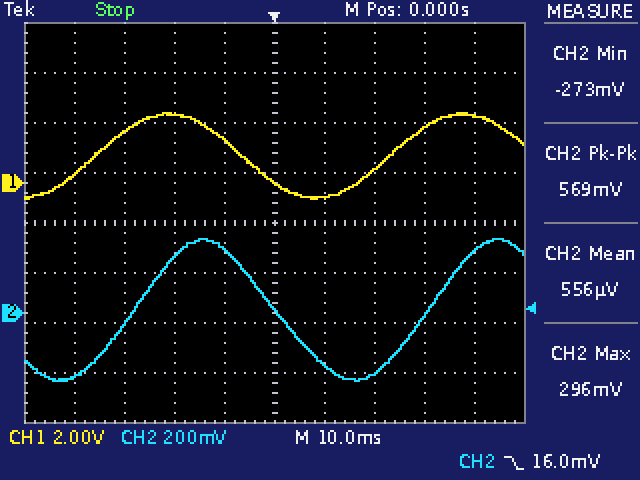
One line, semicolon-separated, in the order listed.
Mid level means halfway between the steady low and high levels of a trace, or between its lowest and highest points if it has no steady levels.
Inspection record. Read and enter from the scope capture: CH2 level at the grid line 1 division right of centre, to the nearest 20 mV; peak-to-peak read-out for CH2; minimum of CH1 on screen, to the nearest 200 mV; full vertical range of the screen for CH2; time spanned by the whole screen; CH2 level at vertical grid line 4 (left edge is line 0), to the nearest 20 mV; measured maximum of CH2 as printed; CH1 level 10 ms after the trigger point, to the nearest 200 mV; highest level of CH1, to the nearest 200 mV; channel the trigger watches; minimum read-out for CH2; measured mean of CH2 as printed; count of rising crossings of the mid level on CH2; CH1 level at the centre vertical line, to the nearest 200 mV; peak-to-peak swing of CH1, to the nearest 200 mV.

-200 mV; 569 mV; -600 mV; 1.6 V; 100 ms; 260 mV; 296 mV; -600 mV; 2.8 V; CH2; -273 mV; 556 µV; 2; 0.0 V; 3.4 V
